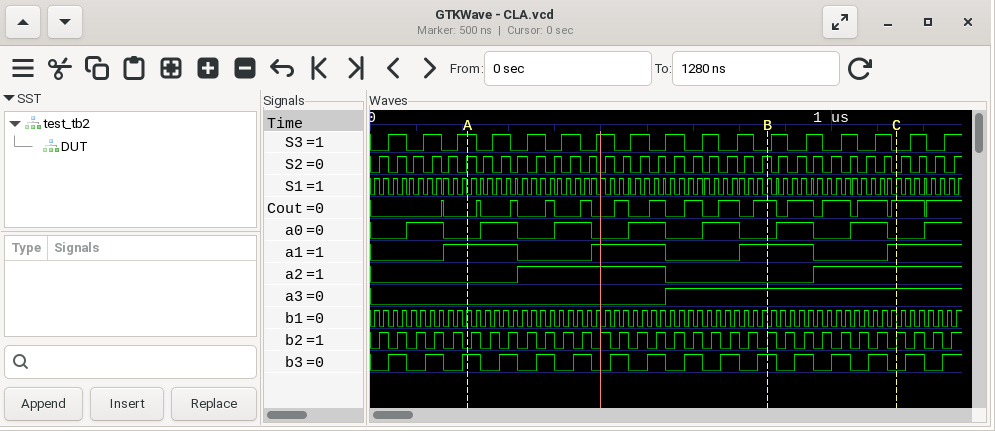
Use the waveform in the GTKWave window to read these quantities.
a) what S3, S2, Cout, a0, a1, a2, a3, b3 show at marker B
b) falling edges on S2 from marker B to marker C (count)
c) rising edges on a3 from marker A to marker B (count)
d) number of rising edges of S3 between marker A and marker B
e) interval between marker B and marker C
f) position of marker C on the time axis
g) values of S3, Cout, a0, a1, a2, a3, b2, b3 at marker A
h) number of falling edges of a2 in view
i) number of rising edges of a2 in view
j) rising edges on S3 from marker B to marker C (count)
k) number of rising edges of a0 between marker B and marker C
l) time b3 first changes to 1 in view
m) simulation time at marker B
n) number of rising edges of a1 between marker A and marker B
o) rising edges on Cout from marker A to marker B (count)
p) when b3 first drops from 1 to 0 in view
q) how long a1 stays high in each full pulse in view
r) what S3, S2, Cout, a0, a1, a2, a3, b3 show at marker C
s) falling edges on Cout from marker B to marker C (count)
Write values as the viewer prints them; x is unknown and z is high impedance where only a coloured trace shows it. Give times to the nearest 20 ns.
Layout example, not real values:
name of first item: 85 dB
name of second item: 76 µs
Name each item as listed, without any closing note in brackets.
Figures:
what S3, S2, Cout, a0, a1, a2, a3, b3 show at marker B: S3=0, S2=1, Cout=1, a0=0, a1=1, a2=0, a3=1, b3=1
falling edges on S2 from marker B to marker C: 8
rising edges on a3 from marker A to marker B: 1
number of rising edges of S3 between marker A and marker B: 8
interval between marker B and marker C: 280 ns
position of marker C on the time axis: 1140 ns
values of S3, Cout, a0, a1, a2, a3, b2, b3 at marker A: S3=1, Cout=0, a0=0, a1=1, a2=0, a3=0, b2=0, b3=1
number of falling edges of a2 in view: 1
number of rising edges of a2 in view: 2
rising edges on S3 from marker B to marker C: 4
number of rising edges of a0 between marker B and marker C: 2
time b3 first changes to 1 in view: 40 ns
simulation time at marker B: 860 ns
number of rising edges of a1 between marker A and marker B: 2
rising edges on Cout from marker A to marker B: 9
when b3 first drops from 1 to 0 in view: 80 ns
how long a1 stays high in each full pulse in view: 160 ns, 160 ns, 160 ns
what S3, S2, Cout, a0, a1, a2, a3, b3 show at marker C: S3=0, S2=0, Cout=1, a0=0, a1=1, a2=1, a3=1, b3=0
falling edges on Cout from marker B to marker C: 4
